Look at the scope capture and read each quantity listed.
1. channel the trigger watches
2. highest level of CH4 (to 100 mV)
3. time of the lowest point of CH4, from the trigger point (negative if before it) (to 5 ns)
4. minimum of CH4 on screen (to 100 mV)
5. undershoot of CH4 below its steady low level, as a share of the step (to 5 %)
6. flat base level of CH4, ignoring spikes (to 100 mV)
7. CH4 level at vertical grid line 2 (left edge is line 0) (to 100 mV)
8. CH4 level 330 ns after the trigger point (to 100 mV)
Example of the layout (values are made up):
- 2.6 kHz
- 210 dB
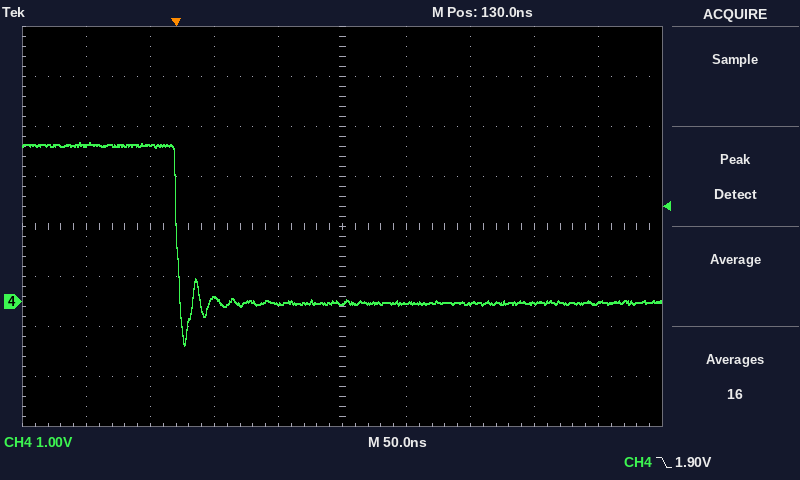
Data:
- CH4
- 3.2 V
- +5 ns
- -900 mV
- 25 %
- 0.0 V
- 3.1 V
- 0.0 V
